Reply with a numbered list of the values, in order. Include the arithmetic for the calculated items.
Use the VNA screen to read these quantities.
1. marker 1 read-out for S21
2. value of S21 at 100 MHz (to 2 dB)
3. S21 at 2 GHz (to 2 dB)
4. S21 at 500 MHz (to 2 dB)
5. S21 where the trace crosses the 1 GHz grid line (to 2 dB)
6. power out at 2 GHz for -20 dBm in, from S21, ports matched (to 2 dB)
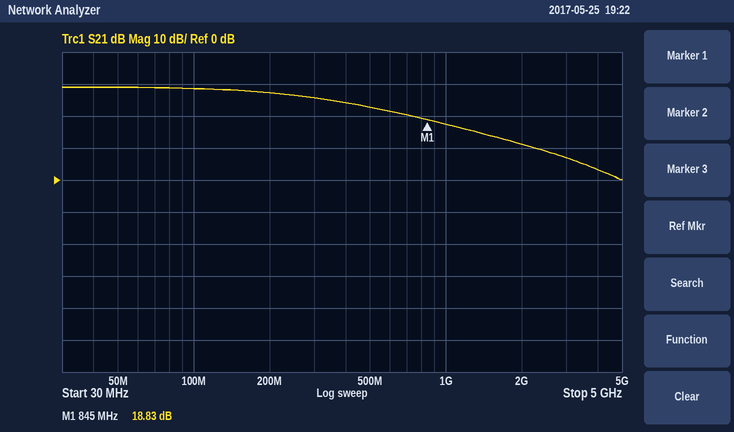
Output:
1. 18.83 dB
2. 28 dB
3. 12 dB
4. 22 dB
5. 18 dB
6. -20 dBm + (12 dB) = -8 dBm
